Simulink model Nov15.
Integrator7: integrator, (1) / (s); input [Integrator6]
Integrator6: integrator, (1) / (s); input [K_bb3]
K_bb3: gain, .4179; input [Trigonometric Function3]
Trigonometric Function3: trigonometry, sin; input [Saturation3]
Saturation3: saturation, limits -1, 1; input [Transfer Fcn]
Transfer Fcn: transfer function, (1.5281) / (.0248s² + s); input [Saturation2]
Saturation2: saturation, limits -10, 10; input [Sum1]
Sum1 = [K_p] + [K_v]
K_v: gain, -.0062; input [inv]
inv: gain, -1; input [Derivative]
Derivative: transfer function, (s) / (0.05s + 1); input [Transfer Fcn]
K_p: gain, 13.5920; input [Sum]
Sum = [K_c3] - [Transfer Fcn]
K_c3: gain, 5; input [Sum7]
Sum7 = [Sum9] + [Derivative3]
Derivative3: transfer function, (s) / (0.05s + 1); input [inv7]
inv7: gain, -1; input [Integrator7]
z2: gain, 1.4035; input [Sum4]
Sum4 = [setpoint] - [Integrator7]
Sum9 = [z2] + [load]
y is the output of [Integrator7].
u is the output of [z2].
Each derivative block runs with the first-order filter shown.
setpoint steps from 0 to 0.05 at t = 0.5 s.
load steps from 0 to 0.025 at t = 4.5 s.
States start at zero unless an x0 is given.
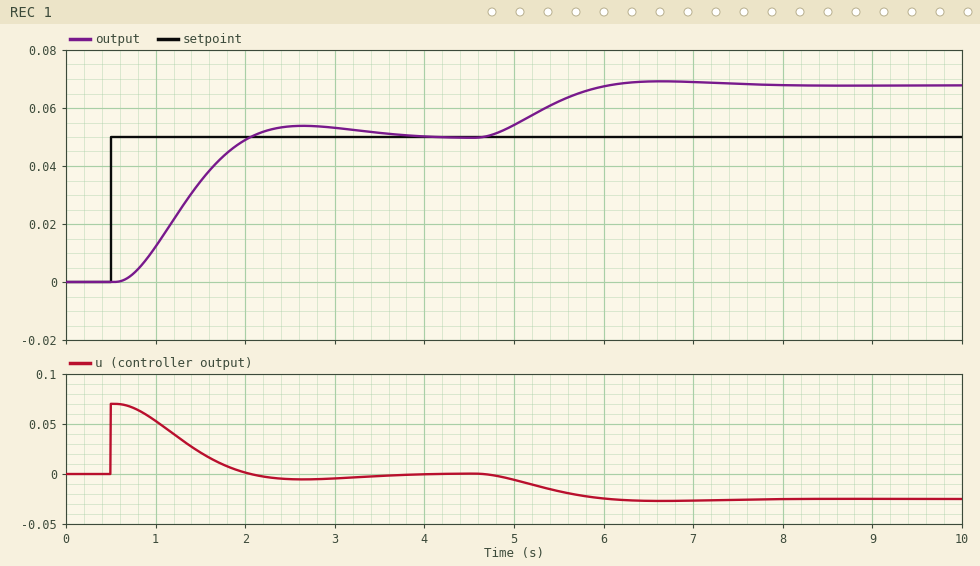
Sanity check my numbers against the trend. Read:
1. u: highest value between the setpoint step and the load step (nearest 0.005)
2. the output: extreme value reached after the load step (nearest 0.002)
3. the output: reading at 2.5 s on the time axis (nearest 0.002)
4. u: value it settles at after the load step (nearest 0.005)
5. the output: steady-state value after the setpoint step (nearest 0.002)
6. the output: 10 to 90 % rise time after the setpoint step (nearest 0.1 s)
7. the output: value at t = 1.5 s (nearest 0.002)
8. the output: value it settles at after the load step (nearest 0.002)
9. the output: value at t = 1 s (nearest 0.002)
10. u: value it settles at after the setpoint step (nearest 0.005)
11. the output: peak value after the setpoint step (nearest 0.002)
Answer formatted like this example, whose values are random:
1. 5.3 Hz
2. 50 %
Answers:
1. 0.070
2. 0.070
3. 0.054
4. -0.025
5. 0.050
6. 1.0 s
7. 0.034
8. 0.068
9. 0.012
10. 0.000
11. 0.054
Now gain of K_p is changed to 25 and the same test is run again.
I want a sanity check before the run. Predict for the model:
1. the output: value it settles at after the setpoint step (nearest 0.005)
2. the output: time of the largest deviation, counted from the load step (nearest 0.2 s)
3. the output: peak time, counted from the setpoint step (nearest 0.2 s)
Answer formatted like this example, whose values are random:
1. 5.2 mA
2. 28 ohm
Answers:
1. 0.050
2. 2.2 s
3. 2.2 s
